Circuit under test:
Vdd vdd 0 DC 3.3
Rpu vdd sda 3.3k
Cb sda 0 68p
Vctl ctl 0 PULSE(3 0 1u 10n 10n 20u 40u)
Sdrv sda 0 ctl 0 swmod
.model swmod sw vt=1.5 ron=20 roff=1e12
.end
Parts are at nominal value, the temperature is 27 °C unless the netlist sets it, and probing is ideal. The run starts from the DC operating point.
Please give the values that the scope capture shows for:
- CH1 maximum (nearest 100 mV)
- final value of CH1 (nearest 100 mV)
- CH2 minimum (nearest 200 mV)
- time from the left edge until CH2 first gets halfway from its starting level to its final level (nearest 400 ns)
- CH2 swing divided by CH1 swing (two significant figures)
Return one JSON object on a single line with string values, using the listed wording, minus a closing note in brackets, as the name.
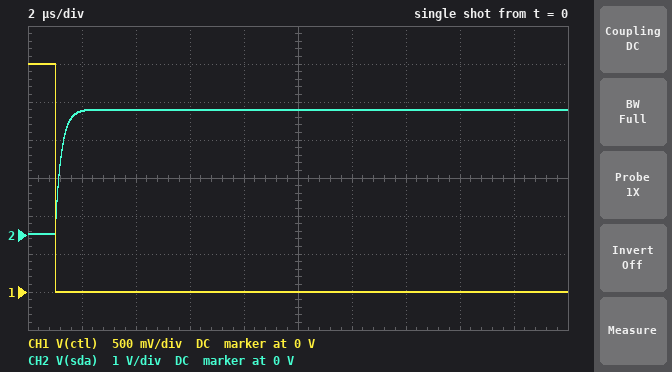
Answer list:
{"CH1 maximum": "3.0 V", "final value of CH1": "0 V", "CH2 minimum": "0 V", "time from the left edge until CH2 first gets halfway from its starting level to its final level": "1.2 µs", "CH2 swing divided by CH1 swing": "1.1"}
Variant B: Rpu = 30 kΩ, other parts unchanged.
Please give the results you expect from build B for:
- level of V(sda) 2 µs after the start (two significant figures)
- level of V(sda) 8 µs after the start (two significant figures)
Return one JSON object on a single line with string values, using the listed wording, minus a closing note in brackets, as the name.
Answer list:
{"level of V(sda) 2 µs after the start": "1.3 V", "level of V(sda) 8 µs after the start": "3.2 V"}
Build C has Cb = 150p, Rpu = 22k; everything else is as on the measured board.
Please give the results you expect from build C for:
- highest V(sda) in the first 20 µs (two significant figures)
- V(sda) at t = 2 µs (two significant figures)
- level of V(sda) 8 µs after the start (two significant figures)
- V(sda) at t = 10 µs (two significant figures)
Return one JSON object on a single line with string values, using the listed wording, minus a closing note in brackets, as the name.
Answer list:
{"highest V(sda) in the first 20 µs": "3.3 V", "V(sda) at t = 2 µs": "860 mV", "level of V(sda) 8 µs after the start": "2.9 V", "V(sda) at t = 10 µs": "3.1 V"}
